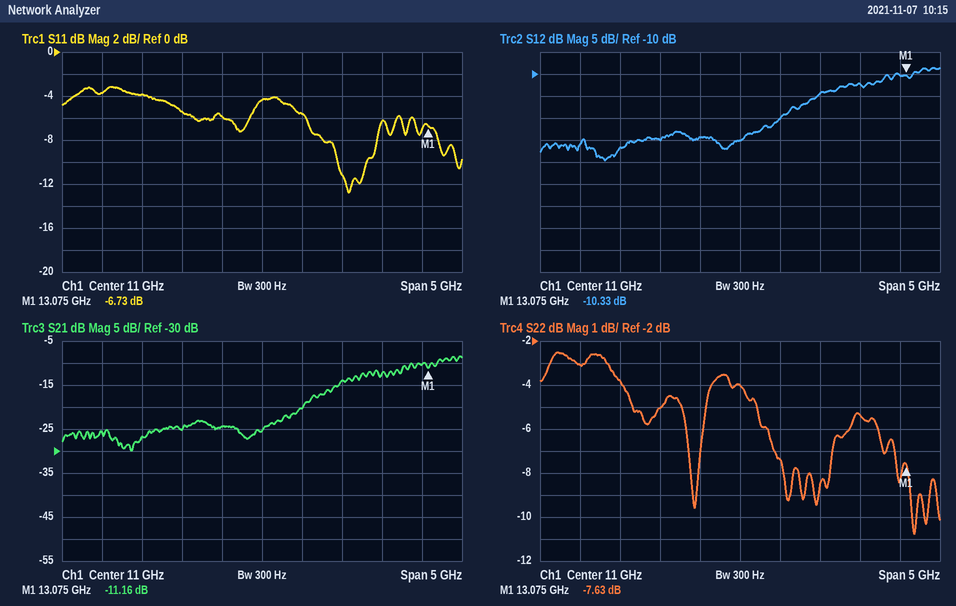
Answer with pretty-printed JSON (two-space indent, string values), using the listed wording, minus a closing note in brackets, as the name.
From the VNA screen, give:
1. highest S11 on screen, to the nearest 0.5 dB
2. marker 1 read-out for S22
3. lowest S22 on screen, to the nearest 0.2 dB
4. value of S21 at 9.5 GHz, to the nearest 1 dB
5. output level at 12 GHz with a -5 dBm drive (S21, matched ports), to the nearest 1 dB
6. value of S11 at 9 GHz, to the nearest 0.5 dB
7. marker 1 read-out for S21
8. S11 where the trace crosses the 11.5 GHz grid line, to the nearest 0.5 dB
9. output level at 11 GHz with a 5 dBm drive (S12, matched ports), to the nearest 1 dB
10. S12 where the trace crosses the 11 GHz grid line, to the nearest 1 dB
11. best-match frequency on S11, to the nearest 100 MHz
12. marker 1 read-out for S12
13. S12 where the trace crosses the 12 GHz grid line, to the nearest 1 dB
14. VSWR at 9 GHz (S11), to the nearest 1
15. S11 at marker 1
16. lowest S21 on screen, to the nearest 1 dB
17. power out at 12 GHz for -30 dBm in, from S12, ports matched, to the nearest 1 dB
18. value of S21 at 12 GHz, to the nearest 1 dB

{
  "highest S11 on screen, to the nearest 0.5 dB": "-3.0 dB",
  "marker 1 read-out for S22": "-7.63 dB",
  "lowest S22 on screen, to the nearest 0.2 dB": "-10.8 dB",
  "value of S21 at 9.5 GHz, to the nearest 1 dB": "-27 dB",
  "output level at 12 GHz with a -5 dBm drive (S21, matched ports), to the nearest 1 dB": "-19 dBm",
  "value of S11 at 9 GHz, to the nearest 0.5 dB": "-3.5 dB",
  "marker 1 read-out for S21": "-11.16 dB",
  "S11 where the trace crosses the 11.5 GHz grid line, to the nearest 0.5 dB": "-5.5 dB",
  "output level at 11 GHz with a 5 dBm drive (S12, matched ports), to the nearest 1 dB": "-20 dBm",
  "S12 where the trace crosses the 11 GHz grid line, to the nearest 1 dB": "-25 dB",
  "best-match frequency on S11, to the nearest 100 MHz": "12.1 GHz",
  "marker 1 read-out for S12": "-10.33 dB",
  "S12 where the trace crosses the 12 GHz grid line, to the nearest 1 dB": "-14 dB",
  "VSWR at 9 GHz (S11), to the nearest 1": "5",
  "S11 at marker 1": "-6.73 dB",
  "lowest S21 on screen, to the nearest 1 dB": "-30 dB",
  "power out at 12 GHz for -30 dBm in, from S12, ports matched, to the nearest 1 dB": "-44 dBm",
  "value of S21 at 12 GHz, to the nearest 1 dB": "-14 dB"
}
